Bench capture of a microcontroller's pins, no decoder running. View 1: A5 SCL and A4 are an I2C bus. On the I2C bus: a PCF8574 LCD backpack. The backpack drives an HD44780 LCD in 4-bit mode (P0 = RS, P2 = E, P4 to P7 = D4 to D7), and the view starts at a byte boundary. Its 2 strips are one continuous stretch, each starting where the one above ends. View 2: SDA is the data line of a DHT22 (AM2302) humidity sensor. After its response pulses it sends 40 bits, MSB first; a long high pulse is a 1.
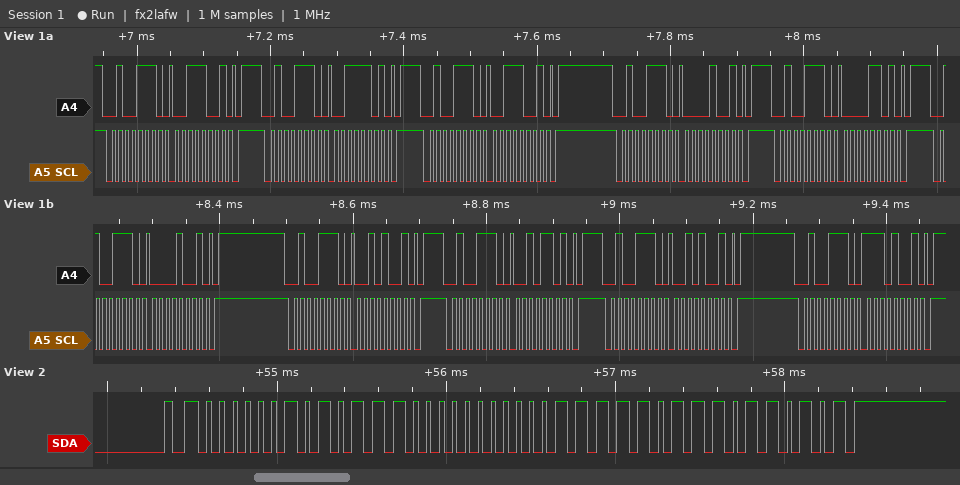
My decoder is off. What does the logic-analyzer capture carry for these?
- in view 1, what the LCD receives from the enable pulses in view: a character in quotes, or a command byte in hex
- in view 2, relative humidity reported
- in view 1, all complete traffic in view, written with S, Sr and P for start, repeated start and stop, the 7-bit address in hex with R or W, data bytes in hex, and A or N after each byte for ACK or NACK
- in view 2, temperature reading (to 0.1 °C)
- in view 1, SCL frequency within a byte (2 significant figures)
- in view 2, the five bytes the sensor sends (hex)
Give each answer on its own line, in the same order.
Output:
'0'
69.6 %
S 27W A 39 A P S 27W A 3D A P S 27W A 39 A P S 27W A 09 A P S 27W A 0D A P S 27W A 09 A P S 27W A 29 A P S 27W A 2D A P S 27W A 29 A P S 27W A E9 A P
25.1 °C
100 kHz
02 B8 00 FB B5
